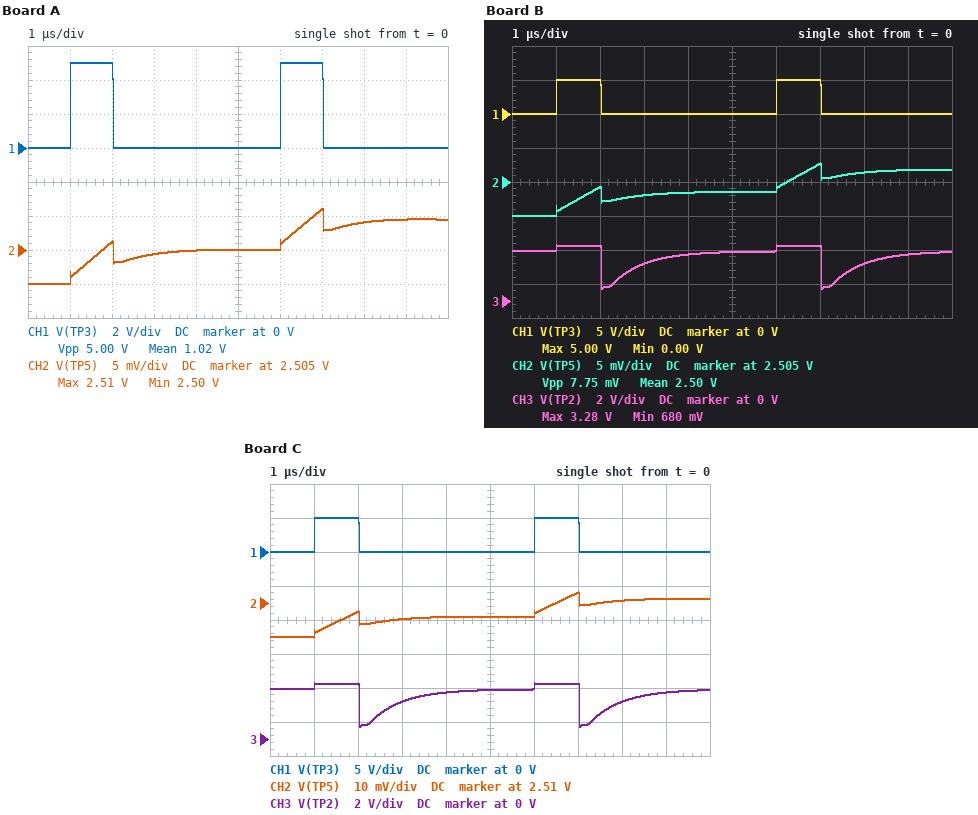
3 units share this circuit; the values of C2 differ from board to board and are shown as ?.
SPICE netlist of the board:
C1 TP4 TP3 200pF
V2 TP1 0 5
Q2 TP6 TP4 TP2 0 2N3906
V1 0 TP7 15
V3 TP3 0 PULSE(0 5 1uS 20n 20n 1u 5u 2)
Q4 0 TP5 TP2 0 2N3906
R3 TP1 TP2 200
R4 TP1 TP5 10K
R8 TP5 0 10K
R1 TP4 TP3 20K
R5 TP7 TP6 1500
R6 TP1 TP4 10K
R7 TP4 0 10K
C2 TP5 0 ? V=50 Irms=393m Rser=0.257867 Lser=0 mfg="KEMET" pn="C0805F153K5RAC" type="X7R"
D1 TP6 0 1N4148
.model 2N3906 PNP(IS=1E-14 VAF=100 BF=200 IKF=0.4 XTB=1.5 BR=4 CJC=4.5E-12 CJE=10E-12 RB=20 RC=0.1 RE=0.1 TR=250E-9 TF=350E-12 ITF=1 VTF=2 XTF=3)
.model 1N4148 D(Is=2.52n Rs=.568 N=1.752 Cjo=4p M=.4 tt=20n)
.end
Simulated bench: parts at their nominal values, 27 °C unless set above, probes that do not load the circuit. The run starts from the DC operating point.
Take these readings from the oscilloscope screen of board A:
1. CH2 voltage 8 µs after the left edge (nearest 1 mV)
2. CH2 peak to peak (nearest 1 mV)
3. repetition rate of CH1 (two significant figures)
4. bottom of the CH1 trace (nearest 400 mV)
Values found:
2.509 V
11 mV
200 kHz
0 V
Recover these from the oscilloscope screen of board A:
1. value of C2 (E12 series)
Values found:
8.2 nF
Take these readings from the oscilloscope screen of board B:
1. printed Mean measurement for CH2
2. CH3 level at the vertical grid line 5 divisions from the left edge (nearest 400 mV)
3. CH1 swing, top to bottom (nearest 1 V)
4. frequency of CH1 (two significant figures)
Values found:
2.50 V
2.8 V
5 V
200 kHz
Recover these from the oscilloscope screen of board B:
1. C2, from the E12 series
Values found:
12 nF
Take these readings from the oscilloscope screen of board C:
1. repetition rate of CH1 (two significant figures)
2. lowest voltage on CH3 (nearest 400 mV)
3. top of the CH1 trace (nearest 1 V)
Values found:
200 kHz
800 mV
5 V
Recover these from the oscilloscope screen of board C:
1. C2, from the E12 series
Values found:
6.8 nF
